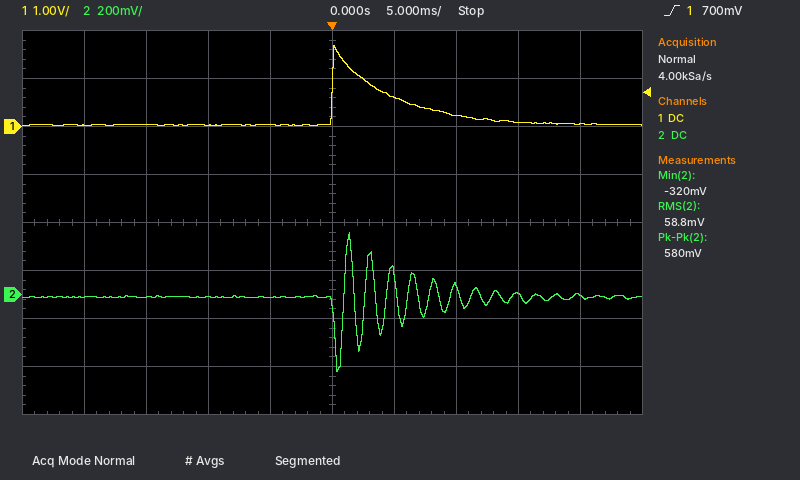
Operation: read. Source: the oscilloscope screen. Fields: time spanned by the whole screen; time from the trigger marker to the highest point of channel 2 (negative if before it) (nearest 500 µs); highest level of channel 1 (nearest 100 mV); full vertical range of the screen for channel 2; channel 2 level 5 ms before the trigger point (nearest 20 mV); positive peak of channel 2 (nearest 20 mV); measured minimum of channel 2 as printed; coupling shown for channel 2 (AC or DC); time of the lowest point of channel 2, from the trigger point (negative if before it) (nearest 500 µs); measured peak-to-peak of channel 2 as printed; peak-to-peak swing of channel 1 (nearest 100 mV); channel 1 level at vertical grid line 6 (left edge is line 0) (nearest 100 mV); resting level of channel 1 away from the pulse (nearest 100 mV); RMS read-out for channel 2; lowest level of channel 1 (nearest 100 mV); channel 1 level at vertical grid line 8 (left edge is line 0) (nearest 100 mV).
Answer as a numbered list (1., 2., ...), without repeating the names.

1. 50 ms
2. +1.5 ms
3. 1.7 V
4. 1.6 V
5. -20 mV
6. 260 mV
7. -320 mV
8. DC
9. +500 µs
10. 580 mV
11. 1.7 V
12. 600 mV
13. 0.0 V
14. 58.8 mV
15. 0.0 V
16. 100 mV
